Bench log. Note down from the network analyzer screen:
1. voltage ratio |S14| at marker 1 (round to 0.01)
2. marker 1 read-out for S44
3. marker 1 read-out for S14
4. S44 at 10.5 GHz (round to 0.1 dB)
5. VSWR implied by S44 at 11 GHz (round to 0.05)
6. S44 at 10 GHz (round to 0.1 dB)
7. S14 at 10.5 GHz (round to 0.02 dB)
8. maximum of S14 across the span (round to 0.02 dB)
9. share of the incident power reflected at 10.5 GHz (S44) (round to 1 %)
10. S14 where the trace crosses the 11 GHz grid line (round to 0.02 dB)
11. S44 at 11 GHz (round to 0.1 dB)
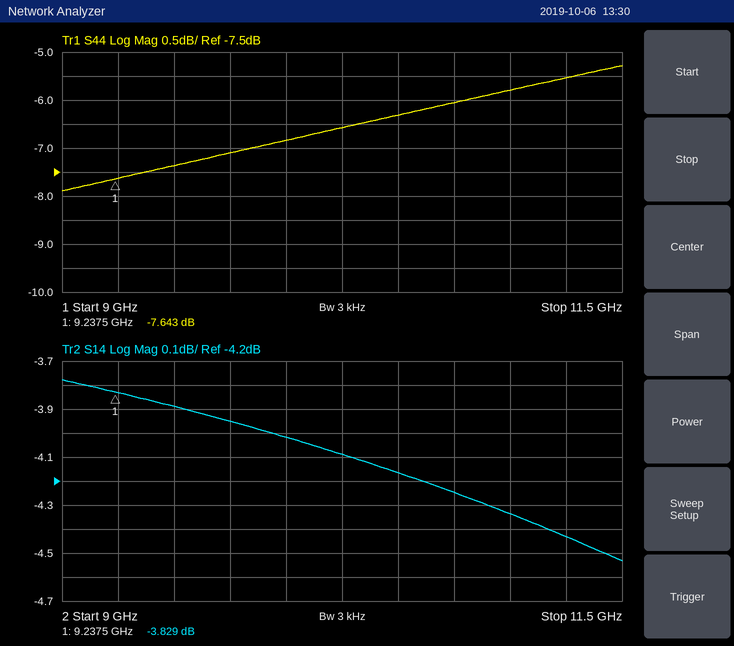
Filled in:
0.64
-7.643 dB
-3.829 dB
-6.3 dB
3.10
-6.8 dB
-4.16 dB
-3.78 dB
23 %
-4.34 dB
-5.8 dB
